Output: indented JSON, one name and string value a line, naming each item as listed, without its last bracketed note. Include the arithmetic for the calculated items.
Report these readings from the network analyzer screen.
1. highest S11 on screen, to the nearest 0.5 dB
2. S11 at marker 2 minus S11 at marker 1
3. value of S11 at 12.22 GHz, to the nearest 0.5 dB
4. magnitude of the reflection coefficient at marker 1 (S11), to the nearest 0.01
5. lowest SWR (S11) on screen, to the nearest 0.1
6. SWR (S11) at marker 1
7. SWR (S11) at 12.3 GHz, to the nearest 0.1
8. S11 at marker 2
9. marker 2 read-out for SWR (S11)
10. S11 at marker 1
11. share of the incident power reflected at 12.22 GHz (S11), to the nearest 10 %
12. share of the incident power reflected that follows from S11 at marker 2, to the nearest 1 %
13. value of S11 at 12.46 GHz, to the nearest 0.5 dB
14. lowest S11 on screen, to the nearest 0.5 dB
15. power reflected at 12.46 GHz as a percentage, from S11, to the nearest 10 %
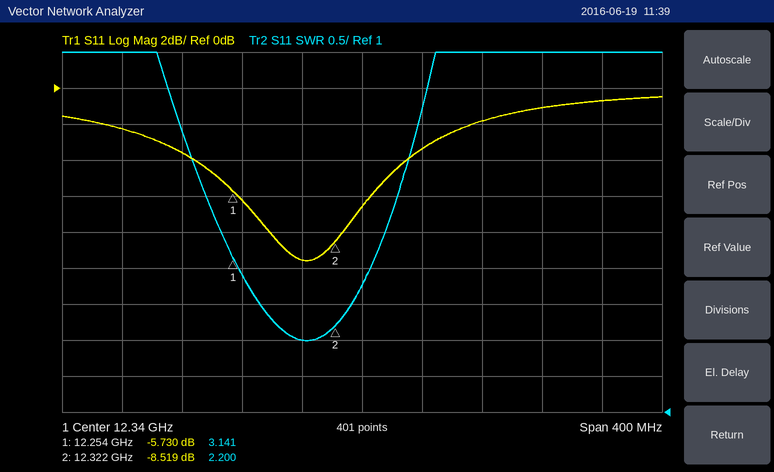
{
  "highest S11 on screen, to the nearest 0.5 dB": "-0.5 dB",
  "S11 at marker 2 minus S11 at marker 1": "-8.519 − (-5.73) = -2.789 dB",
  "value of S11 at 12.22 GHz, to the nearest 0.5 dB": "-3.5 dB",
  "magnitude of the reflection coefficient at marker 1 (S11), to the nearest 0.01": "10^(-5.73/20) ≈ 0.52",
  "lowest SWR (S11) on screen, to the nearest 0.1": "2.0",
  "SWR (S11) at marker 1": "3.141",
  "SWR (S11) at 12.3 GHz, to the nearest 0.1": "2.0",
  "S11 at marker 2": "-8.519 dB",
  "marker 2 read-out for SWR": "2.200",
  "S11 at marker 1": "-5.730 dB",
  "share of the incident power reflected at 12.22 GHz (S11), to the nearest 10 %": "10^(-3.5/10) ≈ 44.7 %, so 40 % to the nearest 10 %",
  "share of the incident power reflected that follows from S11 at marker 2, to the nearest 1 %": "10^(-8.519/10) ≈ 14 %",
  "value of S11 at 12.46 GHz, to the nearest 0.5 dB": "-1.0 dB",
  "lowest S11 on screen, to the nearest 0.5 dB": "-9.5 dB",
  "power reflected at 12.46 GHz as a percentage, from S11, to the nearest 10 %": "10^(-1/10) ≈ 79.4 %, so 80 % to the nearest 10 %"
}
